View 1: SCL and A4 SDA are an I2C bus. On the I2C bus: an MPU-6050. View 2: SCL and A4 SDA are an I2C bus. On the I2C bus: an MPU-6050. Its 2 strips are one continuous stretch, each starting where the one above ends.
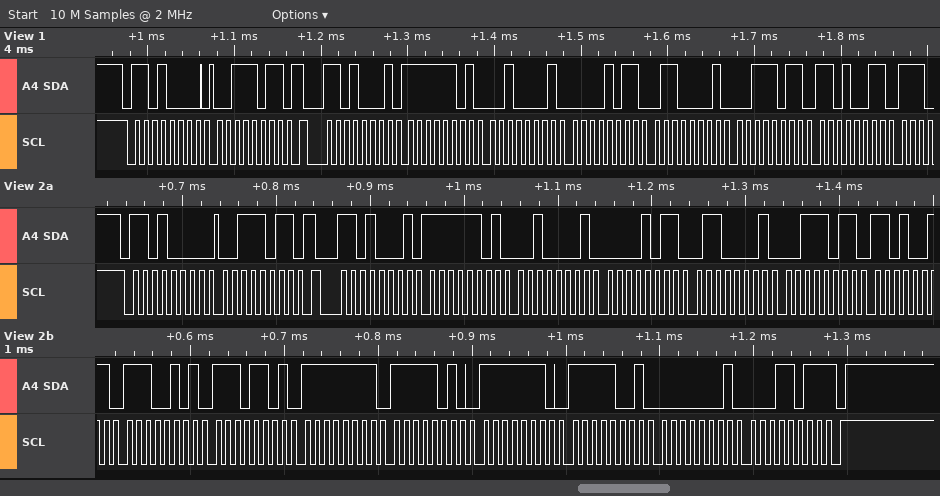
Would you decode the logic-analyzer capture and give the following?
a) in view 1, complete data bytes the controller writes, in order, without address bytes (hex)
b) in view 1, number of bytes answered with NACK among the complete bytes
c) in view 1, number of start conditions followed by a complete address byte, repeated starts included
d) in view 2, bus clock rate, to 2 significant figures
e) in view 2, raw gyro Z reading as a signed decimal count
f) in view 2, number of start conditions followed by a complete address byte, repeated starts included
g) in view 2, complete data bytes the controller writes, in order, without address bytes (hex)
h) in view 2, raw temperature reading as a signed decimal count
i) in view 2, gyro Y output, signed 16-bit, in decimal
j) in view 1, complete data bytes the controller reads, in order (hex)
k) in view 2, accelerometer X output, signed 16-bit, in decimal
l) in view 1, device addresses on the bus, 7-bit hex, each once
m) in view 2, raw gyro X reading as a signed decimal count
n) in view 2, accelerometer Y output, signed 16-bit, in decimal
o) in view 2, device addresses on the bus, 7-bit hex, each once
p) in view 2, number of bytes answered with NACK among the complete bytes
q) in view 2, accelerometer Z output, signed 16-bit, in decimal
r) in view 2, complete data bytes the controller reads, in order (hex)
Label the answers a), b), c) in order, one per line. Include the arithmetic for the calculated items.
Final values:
a) 3B
b) 0
c) 2
d) 100 kHz
e) 0x011B = 283
f) 2
g) 3B
h) 0xE5ED = -6675
i) 0xFEF9 = -263
j) FD 21 0B 61 3B D3
k) 0xFD21 = -735
l) 0x68
m) 0xFFFA = -6
n) 0x0B61 = 2913
o) 0x68
p) 1
q) 0x3BD3 = 15315
r) FD 21 0B 61 3B D3 E5 ED FF FA FE F9 01 1B
